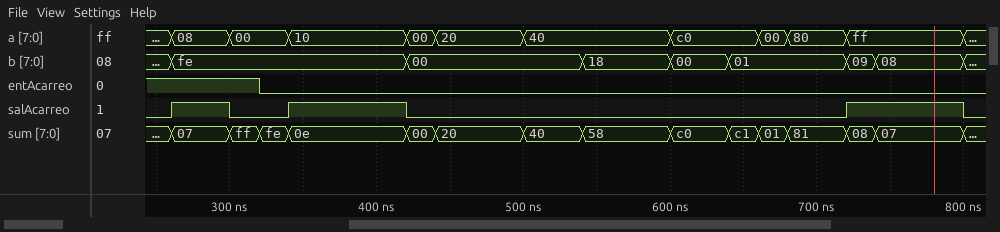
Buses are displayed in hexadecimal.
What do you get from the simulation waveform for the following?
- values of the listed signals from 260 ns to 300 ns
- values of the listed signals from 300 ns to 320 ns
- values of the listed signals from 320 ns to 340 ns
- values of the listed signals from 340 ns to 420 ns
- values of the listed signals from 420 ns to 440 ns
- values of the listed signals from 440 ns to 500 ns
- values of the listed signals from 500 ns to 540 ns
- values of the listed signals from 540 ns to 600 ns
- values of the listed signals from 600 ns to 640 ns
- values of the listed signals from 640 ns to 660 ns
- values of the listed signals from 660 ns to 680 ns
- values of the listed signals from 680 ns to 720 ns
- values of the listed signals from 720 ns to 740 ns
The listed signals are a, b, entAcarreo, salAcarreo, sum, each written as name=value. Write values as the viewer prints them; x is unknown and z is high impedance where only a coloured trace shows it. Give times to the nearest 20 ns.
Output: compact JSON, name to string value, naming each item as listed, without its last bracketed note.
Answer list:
{"values of the listed signals from 260 ns to 300 ns": "a=08, b=fe, entAcarreo=1, salAcarreo=1, sum=07", "values of the listed signals from 300 ns to 320 ns": "a=00, b=fe, entAcarreo=1, salAcarreo=0, sum=ff", "values of the listed signals from 320 ns to 340 ns": "a=00, b=fe, entAcarreo=0, salAcarreo=0, sum=fe", "values of the listed signals from 340 ns to 420 ns": "a=10, b=fe, entAcarreo=0, salAcarreo=1, sum=0e", "values of the listed signals from 420 ns to 440 ns": "a=00, b=00, entAcarreo=0, salAcarreo=0, sum=00", "values of the listed signals from 440 ns to 500 ns": "a=20, b=00, entAcarreo=0, salAcarreo=0, sum=20", "values of the listed signals from 500 ns to 540 ns": "a=40, b=00, entAcarreo=0, salAcarreo=0, sum=40", "values of the listed signals from 540 ns to 600 ns": "a=40, b=18, entAcarreo=0, salAcarreo=0, sum=58", "values of the listed signals from 600 ns to 640 ns": "a=c0, b=00, entAcarreo=0, salAcarreo=0, sum=c0", "values of the listed signals from 640 ns to 660 ns": "a=c0, b=01, entAcarreo=0, salAcarreo=0, sum=c1", "values of the listed signals from 660 ns to 680 ns": "a=00, b=01, entAcarreo=0, salAcarreo=0, sum=01", "values of the listed signals from 680 ns to 720 ns": "a=80, b=01, entAcarreo=0, salAcarreo=0, sum=81", "values of the listed signals from 720 ns to 740 ns": "a=ff, b=09, entAcarreo=0, salAcarreo=1, sum=08"}
